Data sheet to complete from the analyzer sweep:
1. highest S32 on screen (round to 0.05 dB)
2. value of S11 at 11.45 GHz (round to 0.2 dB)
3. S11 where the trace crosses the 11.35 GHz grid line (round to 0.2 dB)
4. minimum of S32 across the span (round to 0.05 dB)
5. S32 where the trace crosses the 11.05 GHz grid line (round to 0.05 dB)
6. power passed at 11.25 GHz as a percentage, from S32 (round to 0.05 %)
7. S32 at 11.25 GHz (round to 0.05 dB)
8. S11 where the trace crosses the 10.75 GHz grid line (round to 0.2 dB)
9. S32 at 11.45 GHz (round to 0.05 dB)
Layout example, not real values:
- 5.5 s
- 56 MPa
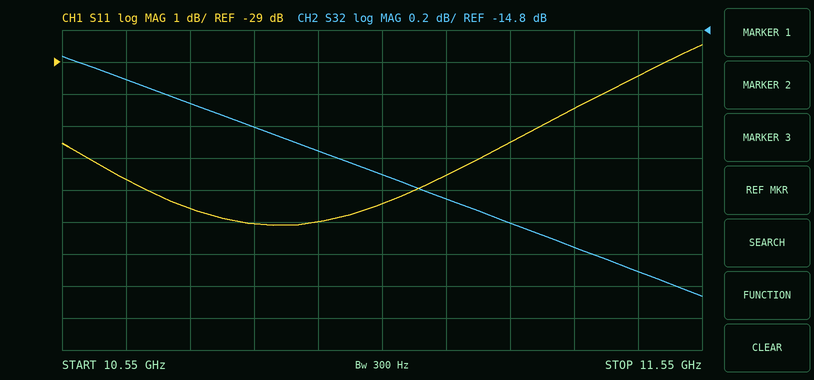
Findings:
- -14.95 dB
- -29.4 dB
- -30.4 dB
- -16.45 dB
- -15.70 dB
- 2.50 %
- -16.00 dB
- -33.6 dB
- -16.30 dB
